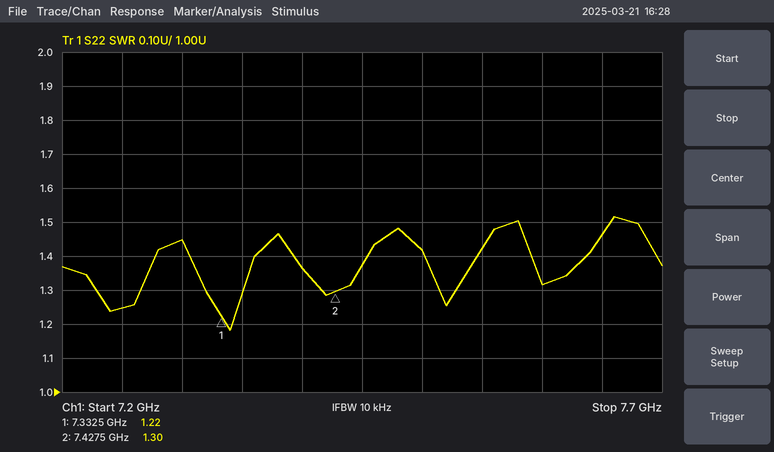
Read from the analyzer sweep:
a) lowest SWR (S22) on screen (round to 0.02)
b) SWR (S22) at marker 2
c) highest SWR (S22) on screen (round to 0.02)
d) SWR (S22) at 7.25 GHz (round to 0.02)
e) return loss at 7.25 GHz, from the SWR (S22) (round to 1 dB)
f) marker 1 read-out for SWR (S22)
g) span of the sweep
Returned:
1.18
1.30
1.52
1.24
19 dB
1.22
500 MHz
